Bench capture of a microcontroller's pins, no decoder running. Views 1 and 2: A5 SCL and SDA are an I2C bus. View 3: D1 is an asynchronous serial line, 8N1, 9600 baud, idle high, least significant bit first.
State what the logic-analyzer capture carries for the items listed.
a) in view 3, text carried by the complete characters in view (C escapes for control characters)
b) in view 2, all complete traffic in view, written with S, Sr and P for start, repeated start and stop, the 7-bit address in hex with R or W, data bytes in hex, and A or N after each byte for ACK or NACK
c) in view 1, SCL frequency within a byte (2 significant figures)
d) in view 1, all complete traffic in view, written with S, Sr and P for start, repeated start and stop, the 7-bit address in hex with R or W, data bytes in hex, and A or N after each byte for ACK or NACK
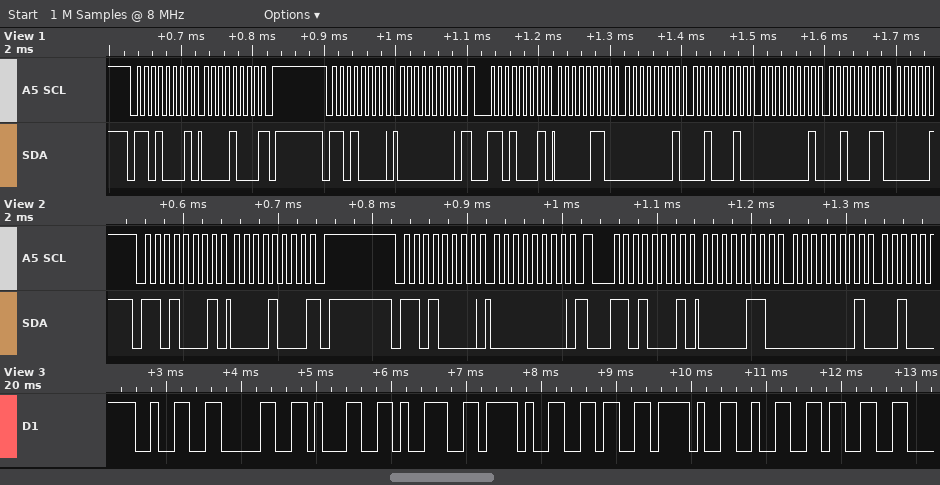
"2019/6/23"
S 68R A 08 N P S 68W A 00 A Sr 68R A 06 A 01 A
100 kHz
S 68R A 08 N P S 68W A 00 A Sr 68R A 06 A 01 A 22 A 01 A 23 A
